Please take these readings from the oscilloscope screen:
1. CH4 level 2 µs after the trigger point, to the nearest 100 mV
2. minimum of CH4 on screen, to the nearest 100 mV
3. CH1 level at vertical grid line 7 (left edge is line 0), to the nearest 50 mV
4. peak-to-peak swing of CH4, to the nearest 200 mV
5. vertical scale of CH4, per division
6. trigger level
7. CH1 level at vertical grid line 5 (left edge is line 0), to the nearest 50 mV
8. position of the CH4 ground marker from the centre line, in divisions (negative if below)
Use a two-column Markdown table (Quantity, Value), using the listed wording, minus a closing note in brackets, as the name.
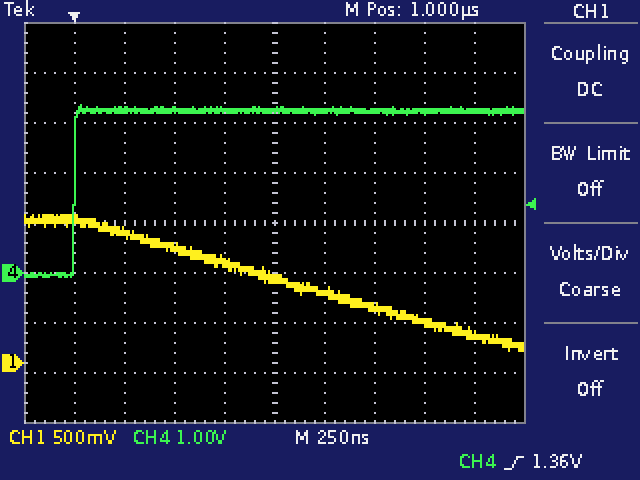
| Quantity | Value |
|---|---|
| CH4 level 2 µs after the trigger point, to the nearest 100 mV | 3.2 V |
| minimum of CH4 on screen, to the nearest 100 mV | -100 mV |
| CH1 level at vertical grid line 7 (left edge is line 0), to the nearest 50 mV | 550 mV |
| peak-to-peak swing of CH4, to the nearest 200 mV | 3.4 V |
| vertical scale of CH4, per division | 1 V |
| trigger level | 1.36 V |
| CH1 level at vertical grid line 5 (left edge is line 0), to the nearest 50 mV | 850 mV |
| position of the CH4 ground marker from the centre line, in divisions | -1.0 div |
